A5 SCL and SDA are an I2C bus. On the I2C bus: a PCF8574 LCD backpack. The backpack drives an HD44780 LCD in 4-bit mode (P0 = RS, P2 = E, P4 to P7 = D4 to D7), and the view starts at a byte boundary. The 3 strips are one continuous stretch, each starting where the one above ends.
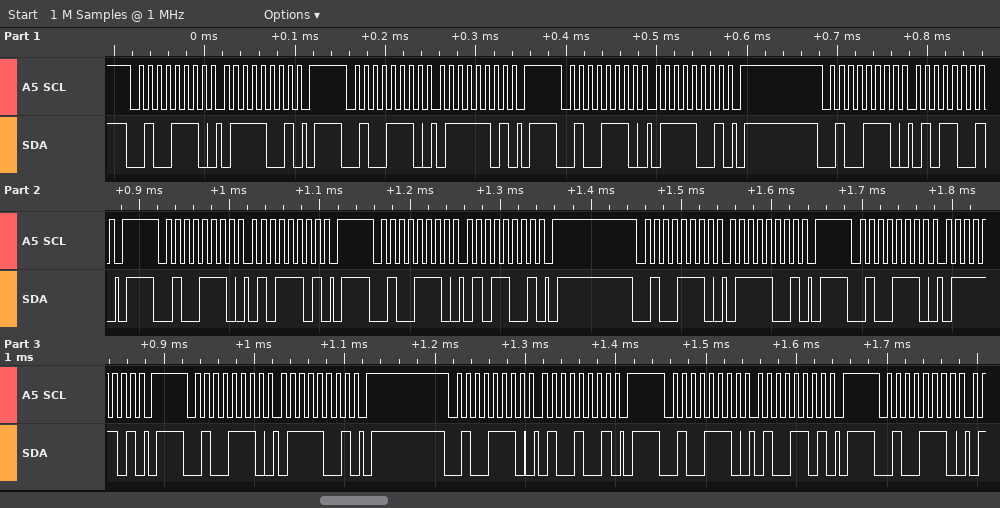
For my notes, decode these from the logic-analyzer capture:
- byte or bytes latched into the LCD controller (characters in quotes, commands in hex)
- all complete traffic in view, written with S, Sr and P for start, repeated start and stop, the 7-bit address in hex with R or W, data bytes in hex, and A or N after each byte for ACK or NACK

'u'
S 27W A 79 A P S 27W A 7D A P S 27W A 79 A P S 27W A 59 A P S 27W A 5D A P S 27W A 59 A P S 27W A 79 A P S 27W A 7D A P S 27W A 79 A P S 27W A 49 A P S 27W A 4D A P S 27W A
